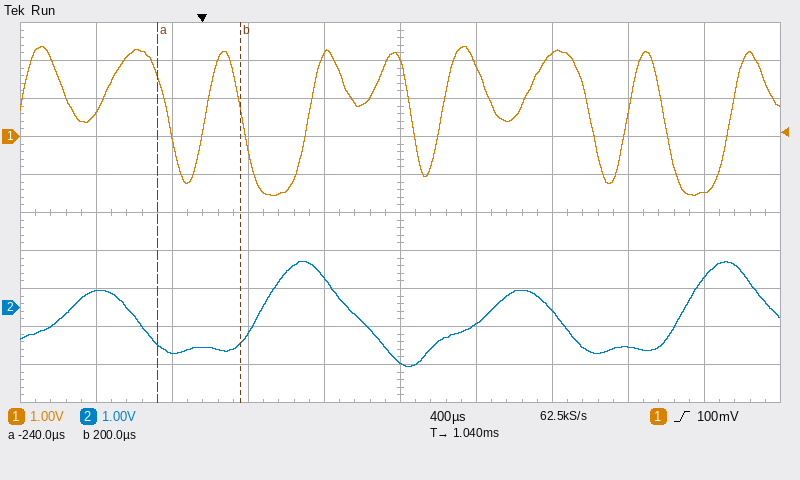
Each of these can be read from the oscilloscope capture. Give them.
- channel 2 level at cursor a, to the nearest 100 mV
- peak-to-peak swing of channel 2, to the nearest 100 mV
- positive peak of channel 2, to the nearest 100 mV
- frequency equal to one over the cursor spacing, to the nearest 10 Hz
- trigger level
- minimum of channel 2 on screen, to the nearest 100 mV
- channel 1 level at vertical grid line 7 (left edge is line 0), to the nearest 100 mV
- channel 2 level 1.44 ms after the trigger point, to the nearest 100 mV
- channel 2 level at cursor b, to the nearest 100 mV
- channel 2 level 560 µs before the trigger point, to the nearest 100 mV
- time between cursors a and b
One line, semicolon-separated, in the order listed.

-1.0 V; 2.8 V; 1.2 V; 2.27 kHz; 100 mV; -1.6 V; 2.2 V; -400 mV; -900 mV; 400 mV; 440 µs
